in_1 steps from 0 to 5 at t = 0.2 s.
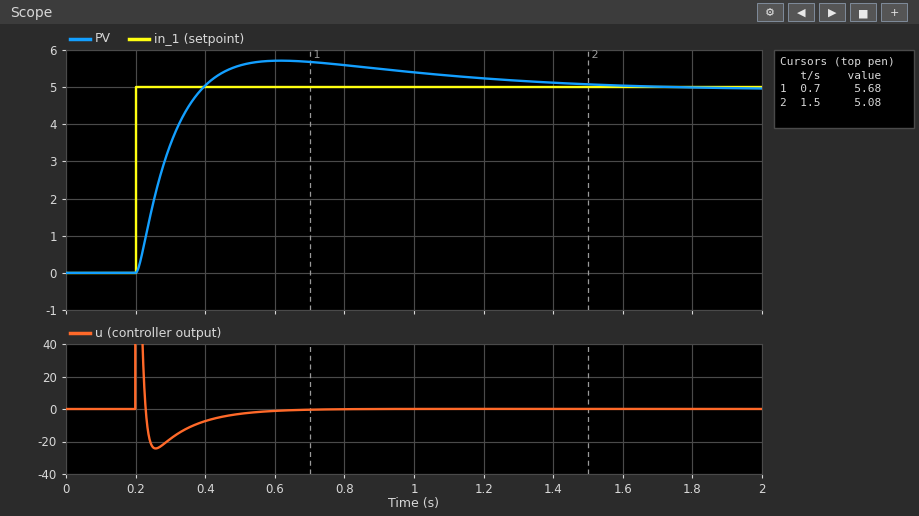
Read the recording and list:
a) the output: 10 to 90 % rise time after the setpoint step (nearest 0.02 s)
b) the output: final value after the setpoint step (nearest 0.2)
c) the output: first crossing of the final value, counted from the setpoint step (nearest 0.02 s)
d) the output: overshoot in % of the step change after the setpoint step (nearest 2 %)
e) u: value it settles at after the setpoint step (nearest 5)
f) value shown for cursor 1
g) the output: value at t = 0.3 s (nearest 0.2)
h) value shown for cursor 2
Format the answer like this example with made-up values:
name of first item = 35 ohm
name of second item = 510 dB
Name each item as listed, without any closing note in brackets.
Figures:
the output: 10 to 90 % rise time after the setpoint step = 0.14 s
the output: final value after the setpoint step = 5.0
the output: first crossing of the final value, counted from the setpoint step = 0.20 s
the output: overshoot in % of the step change after the setpoint step = 14 %
u: value it settles at after the setpoint step = 0
value shown for cursor 1 = 5.68
the output: value at t = 0.3 s = 3.4
value shown for cursor 2 = 5.08
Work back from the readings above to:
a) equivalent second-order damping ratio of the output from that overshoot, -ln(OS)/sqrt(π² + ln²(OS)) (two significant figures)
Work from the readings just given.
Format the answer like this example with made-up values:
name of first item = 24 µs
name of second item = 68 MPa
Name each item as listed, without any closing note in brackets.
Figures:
equivalent second-order damping ratio of the output from that overshoot, -ln(OS)/sqrt(π² + ln²(OS)) = 0.53
